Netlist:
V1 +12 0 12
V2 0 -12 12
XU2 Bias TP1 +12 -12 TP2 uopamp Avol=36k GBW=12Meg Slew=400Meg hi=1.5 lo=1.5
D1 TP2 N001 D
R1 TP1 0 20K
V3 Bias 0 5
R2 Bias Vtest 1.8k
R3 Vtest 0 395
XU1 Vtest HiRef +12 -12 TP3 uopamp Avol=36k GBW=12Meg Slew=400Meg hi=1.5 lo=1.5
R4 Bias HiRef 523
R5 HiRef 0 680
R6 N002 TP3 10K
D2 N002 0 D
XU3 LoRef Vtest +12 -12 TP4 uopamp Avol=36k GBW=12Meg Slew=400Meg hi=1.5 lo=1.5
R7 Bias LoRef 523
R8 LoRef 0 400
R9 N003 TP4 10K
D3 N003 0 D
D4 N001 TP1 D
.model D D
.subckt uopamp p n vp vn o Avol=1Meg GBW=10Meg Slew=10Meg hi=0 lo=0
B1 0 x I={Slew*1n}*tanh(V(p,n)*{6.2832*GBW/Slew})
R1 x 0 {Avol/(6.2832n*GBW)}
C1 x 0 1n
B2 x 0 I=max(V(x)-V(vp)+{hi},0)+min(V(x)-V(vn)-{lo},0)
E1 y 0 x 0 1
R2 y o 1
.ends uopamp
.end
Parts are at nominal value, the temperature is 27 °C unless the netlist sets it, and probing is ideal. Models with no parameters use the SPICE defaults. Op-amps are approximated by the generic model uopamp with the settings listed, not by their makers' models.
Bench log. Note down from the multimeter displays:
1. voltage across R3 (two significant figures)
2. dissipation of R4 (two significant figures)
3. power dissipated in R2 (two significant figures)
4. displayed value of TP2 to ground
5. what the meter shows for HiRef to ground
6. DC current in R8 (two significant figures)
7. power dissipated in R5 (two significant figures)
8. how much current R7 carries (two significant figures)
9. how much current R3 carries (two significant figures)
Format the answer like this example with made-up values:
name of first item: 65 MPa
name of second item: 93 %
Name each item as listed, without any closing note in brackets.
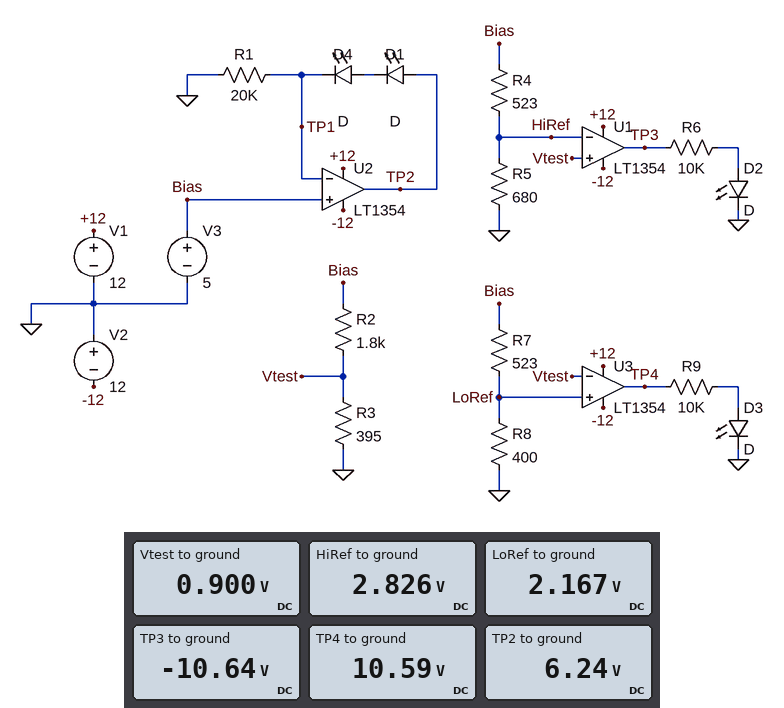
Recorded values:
voltage across R3: 900 mV
dissipation of R4: 9.0 mW
power dissipated in R2: 9.3 mW
displayed value of TP2 to ground: 6.24 V
what the meter shows for HiRef to ground: 2.826 V
DC current in R8: 5.4 mA
power dissipated in R5: 12 mW
how much current R7 carries: 5.4 mA
how much current R3 carries: 2.3 mA
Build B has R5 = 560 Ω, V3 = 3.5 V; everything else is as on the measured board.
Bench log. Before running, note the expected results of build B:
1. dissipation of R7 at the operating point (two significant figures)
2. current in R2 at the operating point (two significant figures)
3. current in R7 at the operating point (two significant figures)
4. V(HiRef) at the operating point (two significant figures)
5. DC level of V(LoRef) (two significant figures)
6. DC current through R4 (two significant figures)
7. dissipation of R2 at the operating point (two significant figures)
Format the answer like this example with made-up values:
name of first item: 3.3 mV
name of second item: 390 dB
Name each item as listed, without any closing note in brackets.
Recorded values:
dissipation of R7 at the operating point: 7.5 mW
current in R2 at the operating point: 1.6 mA
current in R7 at the operating point: 3.8 mA
V(HiRef) at the operating point: 1.8 V
DC level of V(LoRef): 1.5 V
DC current through R4: 3.2 mA
dissipation of R2 at the operating point: 4.6 mW
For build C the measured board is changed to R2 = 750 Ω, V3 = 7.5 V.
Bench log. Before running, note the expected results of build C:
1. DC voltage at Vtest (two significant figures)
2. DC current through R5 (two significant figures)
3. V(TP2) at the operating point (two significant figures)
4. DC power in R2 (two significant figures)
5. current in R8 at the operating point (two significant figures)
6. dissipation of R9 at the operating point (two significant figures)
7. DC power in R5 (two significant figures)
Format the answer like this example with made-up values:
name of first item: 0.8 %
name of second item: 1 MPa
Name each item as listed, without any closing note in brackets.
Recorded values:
DC voltage at Vtest: 2.6 V
DC current through R5: 6.2 mA
V(TP2) at the operating point: 8.8 V
DC power in R2: 32 mW
current in R8 at the operating point: 8.1 mA
dissipation of R9 at the operating point: 9.8 mW
DC power in R5: 26 mW
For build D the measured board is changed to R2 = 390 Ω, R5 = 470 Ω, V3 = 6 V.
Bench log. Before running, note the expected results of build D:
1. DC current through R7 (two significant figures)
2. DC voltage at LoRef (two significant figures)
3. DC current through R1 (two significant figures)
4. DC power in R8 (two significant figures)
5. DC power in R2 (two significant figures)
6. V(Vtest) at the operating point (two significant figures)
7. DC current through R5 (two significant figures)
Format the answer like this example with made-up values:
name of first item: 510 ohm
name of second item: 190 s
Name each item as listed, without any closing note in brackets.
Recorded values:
DC current through R7: 6.5 mA
DC voltage at LoRef: 2.6 V
DC current through R1: 300 µA
DC power in R8: 17 mW
DC power in R2: 23 mW
V(Vtest) at the operating point: 3.0 V
DC current through R5: 6.0 mA
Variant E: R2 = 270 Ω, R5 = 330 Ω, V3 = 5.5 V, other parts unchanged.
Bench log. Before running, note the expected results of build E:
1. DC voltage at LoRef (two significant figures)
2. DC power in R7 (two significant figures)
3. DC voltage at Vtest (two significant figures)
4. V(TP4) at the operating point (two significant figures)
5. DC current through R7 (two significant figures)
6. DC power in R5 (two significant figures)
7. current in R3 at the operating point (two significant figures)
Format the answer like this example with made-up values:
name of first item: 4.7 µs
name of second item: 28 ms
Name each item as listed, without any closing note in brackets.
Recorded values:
DC voltage at LoRef: 2.4 V
DC power in R7: 19 mW
DC voltage at Vtest: 3.3 V
V(TP4) at the operating point: -11 V
DC current through R7: 6.0 mA
DC power in R5: 14 mW
current in R3 at the operating point: 8.3 mA
